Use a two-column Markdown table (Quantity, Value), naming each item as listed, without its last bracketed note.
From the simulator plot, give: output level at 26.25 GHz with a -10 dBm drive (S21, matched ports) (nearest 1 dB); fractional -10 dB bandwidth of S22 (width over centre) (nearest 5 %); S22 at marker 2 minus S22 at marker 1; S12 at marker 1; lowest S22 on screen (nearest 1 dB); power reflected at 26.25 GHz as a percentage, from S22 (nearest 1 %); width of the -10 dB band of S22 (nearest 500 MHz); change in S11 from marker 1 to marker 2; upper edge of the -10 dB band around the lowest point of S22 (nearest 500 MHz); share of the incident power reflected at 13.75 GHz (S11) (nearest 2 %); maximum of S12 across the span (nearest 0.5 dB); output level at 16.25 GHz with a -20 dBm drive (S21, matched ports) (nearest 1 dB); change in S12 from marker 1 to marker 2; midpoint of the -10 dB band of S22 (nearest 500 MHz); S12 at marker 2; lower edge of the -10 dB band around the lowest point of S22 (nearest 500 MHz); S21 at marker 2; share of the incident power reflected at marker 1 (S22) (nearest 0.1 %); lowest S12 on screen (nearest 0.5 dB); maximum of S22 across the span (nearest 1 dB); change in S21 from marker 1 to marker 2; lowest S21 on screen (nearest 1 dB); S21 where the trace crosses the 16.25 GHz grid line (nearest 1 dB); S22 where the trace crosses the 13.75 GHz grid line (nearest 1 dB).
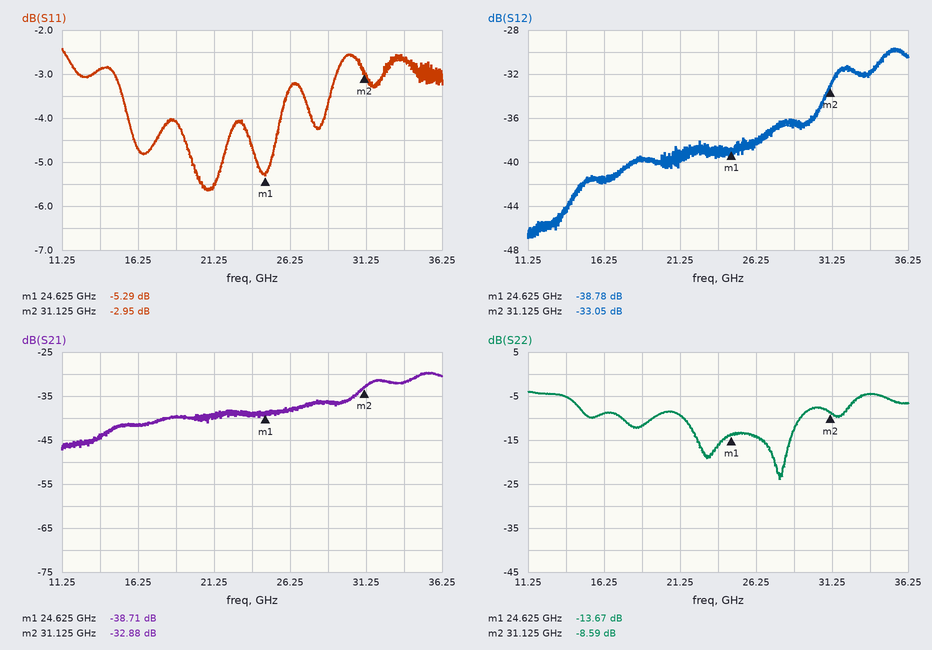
| Quantity | Value |
|---|---|
| output level at 26.25 GHz with a -10 dBm drive (S21, matched ports) | -48 dBm |
| fractional -10 dB bandwidth of S22 (width over centre) | 30 % |
| S22 at marker 2 minus S22 at marker 1 | 5.08 dB |
| S12 at marker 1 | -38.78 dB |
| lowest S22 on screen | -24 dB |
| power reflected at 26.25 GHz as a percentage, from S22 | 4 % |
| width of the -10 dB band of S22 | 7.5 GHz |
| change in S11 from marker 1 to marker 2 | 2.34 dB |
| upper edge of the -10 dB band around the lowest point of S22 | 29.0 GHz |
| share of the incident power reflected at 13.75 GHz (S11) | 52 % |
| maximum of S12 across the span | -29.5 dB |
| output level at 16.25 GHz with a -20 dBm drive (S21, matched ports) | -62 dBm |
| change in S12 from marker 1 to marker 2 | 5.73 dB |
| midpoint of the -10 dB band of S22 | 25.5 GHz |
| S12 at marker 2 | -33.05 dB |
| lower edge of the -10 dB band around the lowest point of S22 | 21.5 GHz |
| S21 at marker 2 | -32.88 dB |
| share of the incident power reflected at marker 1 (S22) | 4.3 % |
| lowest S12 on screen | -47.0 dB |
| maximum of S22 across the span | -4 dB |
| change in S21 from marker 1 to marker 2 | 5.83 dB |
| lowest S21 on screen | -47 dB |
| S21 where the trace crosses the 16.25 GHz grid line | -42 dB |
| S22 where the trace crosses the 13.75 GHz grid line | -5 dB |
